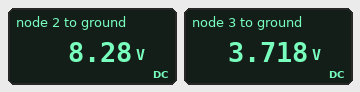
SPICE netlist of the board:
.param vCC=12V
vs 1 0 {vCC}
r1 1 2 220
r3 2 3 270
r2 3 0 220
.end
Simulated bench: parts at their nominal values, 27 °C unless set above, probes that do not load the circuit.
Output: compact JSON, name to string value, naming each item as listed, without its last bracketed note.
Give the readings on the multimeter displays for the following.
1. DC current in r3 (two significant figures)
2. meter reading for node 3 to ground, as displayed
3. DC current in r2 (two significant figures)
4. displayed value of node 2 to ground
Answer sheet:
{"DC current in r3": "17 mA", "meter reading for node 3 to ground, as displayed": "3.718 V", "DC current in r2": "17 mA", "displayed value of node 2 to ground": "8.28 V"}
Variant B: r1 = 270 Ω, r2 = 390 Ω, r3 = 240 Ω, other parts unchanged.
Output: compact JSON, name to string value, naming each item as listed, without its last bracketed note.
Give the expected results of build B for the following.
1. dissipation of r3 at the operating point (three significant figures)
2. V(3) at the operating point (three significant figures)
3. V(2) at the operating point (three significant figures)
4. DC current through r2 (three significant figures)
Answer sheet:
{"dissipation of r3 at the operating point": "42.7 mW", "V(3) at the operating point": "5.20 V", "V(2) at the operating point": "8.40 V", "DC current through r2": "13.3 mA"}
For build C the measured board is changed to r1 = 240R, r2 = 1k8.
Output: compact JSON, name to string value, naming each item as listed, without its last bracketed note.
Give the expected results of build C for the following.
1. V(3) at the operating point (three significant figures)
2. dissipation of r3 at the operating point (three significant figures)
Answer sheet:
{"V(3) at the operating point": "9.35 V", "dissipation of r3 at the operating point": "7.29 mW"}
